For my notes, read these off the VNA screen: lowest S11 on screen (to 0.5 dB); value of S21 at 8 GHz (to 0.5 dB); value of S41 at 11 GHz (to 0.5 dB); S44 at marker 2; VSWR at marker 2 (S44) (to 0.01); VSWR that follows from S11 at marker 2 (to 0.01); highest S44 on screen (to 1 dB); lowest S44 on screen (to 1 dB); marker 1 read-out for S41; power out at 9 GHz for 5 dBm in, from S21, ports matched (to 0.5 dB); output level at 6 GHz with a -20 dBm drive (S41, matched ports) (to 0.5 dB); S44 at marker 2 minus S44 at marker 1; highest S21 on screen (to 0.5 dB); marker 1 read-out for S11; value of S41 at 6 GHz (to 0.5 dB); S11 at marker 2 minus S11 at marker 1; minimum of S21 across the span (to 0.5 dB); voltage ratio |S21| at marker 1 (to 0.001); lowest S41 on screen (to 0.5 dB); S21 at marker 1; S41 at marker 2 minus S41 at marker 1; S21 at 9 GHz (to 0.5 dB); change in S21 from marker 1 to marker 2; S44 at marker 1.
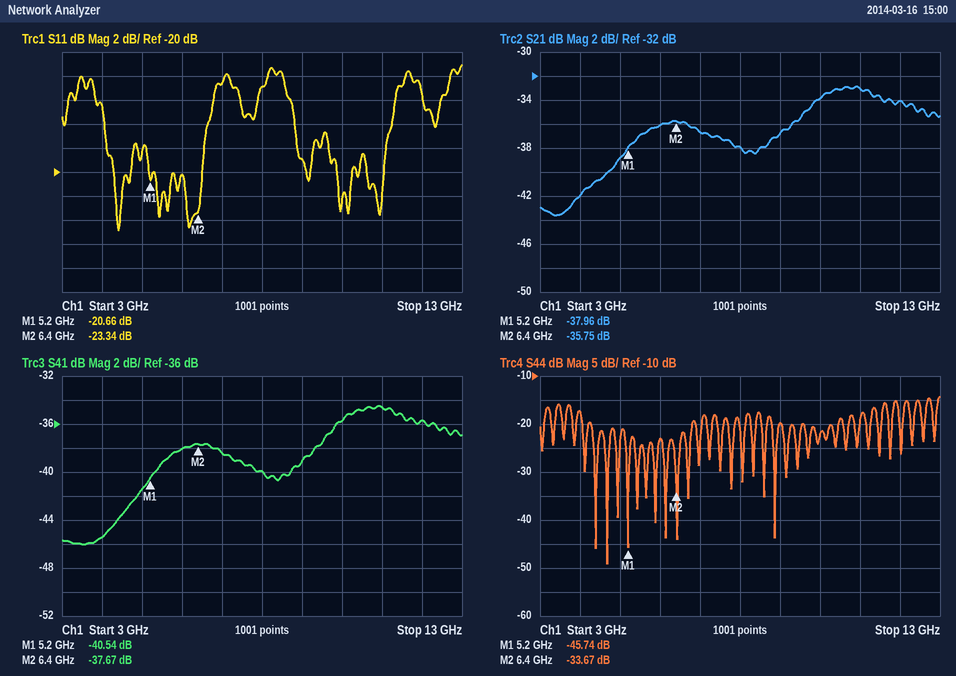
-25.0 dB
-38.0 dB
-34.5 dB
-33.67 dB
1.04
1.15
-14 dB
-49 dB
-40.54 dB
-32.0 dBm
-58.0 dBm
12.07 dB
-33.0 dB
-20.66 dB
-38.0 dB
-2.68 dB
-43.5 dB
0.013
-46.0 dB
-37.96 dB
2.87 dB
-37.0 dB
2.21 dB
-45.74 dB
